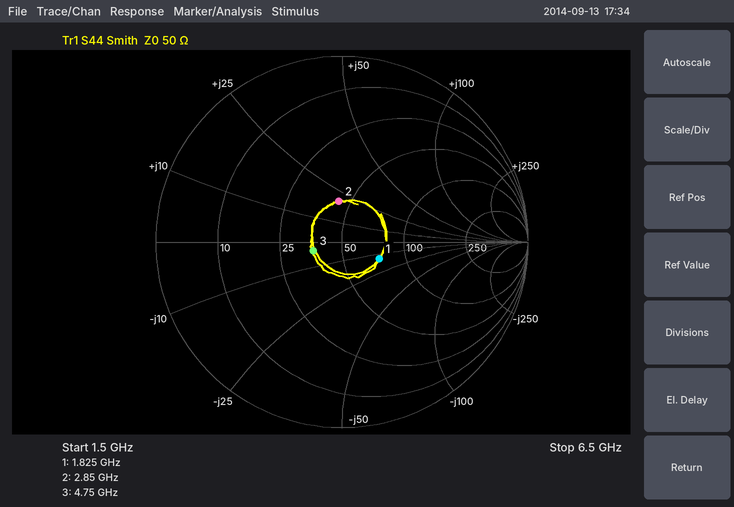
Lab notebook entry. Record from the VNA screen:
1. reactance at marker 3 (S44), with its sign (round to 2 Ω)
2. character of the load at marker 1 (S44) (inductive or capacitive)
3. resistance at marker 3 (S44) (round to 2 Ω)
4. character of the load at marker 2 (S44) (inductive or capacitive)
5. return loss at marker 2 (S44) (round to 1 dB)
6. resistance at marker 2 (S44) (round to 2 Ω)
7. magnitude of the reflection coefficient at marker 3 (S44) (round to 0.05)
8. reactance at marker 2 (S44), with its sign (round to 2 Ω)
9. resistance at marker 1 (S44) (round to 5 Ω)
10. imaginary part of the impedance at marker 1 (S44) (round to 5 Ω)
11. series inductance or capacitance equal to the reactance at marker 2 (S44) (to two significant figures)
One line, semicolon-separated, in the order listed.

-4 Ω; capacitive; 36 Ω; inductive; 13 dB; 44 Ω; 0.15; +20 Ω; 75 Ω; -15 Ω; 1.1 nH
